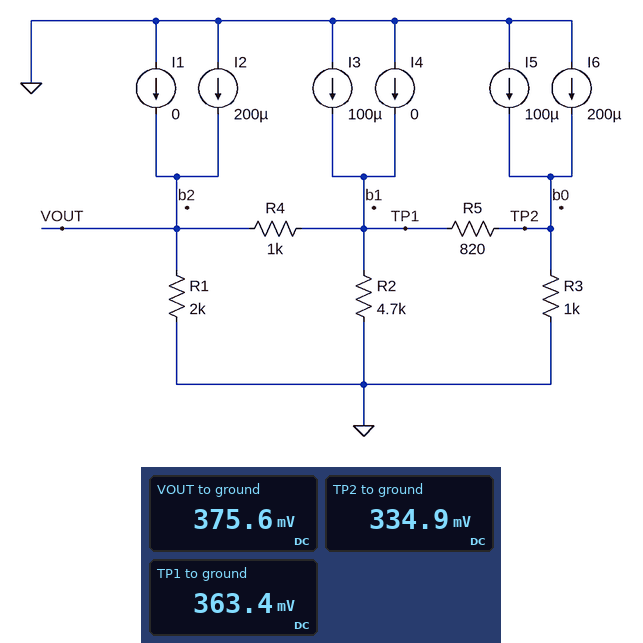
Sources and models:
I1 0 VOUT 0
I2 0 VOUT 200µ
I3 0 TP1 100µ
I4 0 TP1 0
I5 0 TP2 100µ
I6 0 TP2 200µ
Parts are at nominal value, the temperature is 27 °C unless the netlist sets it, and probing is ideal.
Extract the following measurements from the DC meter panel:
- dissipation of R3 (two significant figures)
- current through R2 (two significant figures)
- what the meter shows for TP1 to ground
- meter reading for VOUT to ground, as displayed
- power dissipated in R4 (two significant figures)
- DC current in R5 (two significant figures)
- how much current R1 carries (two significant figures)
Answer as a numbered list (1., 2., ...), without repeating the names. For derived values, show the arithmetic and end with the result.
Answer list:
1. (334.9 mV)^2 / 1 kΩ = 110 µW
2. (363.4 mV) / 4.7 kΩ = 77 µA
3. 363.4 mV
4. 375.6 mV
5. (375.6 mV - 363.4 mV)^2 / 1 kΩ = 150 nW
6. (363.4 mV - 334.9 mV) / 820 Ω = 35 µA
7. (375.6 mV) / 2 kΩ = 190 µA
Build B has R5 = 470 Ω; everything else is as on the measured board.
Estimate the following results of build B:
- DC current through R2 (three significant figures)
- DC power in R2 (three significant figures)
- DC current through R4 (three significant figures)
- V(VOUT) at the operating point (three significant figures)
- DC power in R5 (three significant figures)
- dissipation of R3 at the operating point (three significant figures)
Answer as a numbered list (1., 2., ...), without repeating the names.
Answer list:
1. 75.9 µA
2. 27.1 µW
3. 14.4 µA
4. 371 mV
5. 699 nW
6. 115 µW
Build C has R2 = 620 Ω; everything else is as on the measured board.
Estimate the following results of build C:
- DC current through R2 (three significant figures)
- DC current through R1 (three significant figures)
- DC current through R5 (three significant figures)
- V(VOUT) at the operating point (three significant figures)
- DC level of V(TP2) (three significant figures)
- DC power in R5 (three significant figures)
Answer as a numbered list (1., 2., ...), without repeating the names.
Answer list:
1. 257 µA
2. 120 µA
3. 77.2 µA
4. 240 mV
5. 223 mV
6. 4.88 µW
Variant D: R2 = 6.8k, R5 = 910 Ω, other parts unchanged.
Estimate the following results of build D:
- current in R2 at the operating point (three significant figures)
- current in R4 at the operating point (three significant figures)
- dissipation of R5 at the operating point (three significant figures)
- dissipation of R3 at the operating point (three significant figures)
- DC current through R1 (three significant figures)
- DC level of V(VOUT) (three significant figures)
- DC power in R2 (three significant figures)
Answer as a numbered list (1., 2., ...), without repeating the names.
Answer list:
1. 57.2 µA
2. 3.71 µA
3. 1.97 µW
4. 120 µW
5. 196 µA
6. 393 mV
7. 22.2 µW
